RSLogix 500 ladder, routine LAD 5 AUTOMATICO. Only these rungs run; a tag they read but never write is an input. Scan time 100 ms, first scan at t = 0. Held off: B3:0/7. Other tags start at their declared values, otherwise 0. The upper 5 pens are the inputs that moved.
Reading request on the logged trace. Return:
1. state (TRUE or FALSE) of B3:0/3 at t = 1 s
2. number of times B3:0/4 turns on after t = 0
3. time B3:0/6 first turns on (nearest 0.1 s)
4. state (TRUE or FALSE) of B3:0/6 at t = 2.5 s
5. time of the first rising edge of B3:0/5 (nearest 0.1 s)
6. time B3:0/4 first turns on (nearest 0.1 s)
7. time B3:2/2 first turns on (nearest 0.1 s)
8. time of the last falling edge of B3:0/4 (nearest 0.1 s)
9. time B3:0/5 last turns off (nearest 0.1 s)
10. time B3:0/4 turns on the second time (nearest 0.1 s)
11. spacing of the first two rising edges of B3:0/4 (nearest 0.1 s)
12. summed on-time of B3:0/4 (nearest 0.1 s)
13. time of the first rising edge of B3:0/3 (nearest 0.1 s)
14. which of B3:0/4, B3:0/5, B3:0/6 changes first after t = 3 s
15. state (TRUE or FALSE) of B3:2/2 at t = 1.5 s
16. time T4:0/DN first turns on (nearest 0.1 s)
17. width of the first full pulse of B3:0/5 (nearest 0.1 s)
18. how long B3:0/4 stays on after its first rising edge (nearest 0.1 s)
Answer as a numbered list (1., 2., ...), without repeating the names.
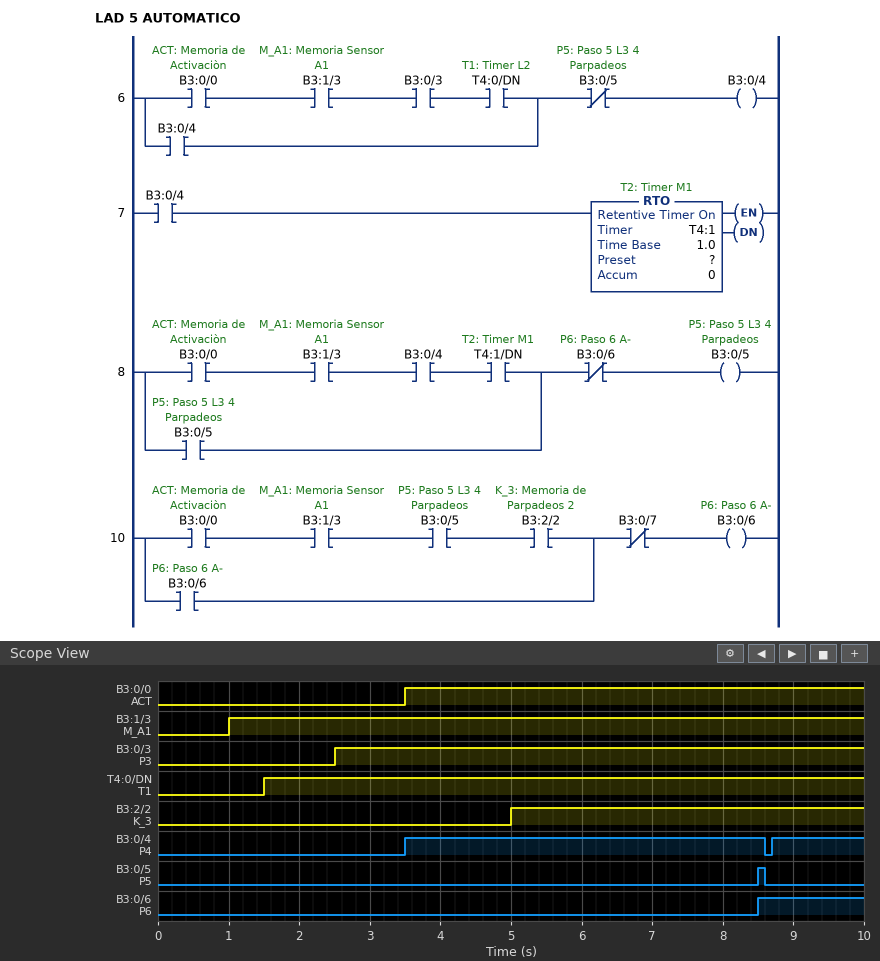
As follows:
1. FALSE
2. 2
3. 8.5 s
4. FALSE
5. 8.5 s
6. 3.5 s
7. 5.0 s
8. 8.6 s
9. 8.6 s
10. 8.7 s
11. 5.2 s
12. 6.4 s
13. 2.5 s
14. B3:0/4
15. FALSE
16. 1.5 s
17. 0.1 s
18. 5.1 s
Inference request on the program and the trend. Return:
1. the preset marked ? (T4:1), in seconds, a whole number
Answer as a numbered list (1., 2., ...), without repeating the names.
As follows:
1. 5 s
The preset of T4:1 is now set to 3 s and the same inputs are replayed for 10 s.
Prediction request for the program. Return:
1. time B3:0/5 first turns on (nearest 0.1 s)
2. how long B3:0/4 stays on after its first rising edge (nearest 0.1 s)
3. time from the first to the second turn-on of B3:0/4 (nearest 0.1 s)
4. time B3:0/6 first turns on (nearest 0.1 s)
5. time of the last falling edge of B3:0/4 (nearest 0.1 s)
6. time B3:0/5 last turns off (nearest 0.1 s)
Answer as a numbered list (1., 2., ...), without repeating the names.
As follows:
1. 6.5 s
2. 3.1 s
3. 3.2 s
4. 6.5 s
5. 6.6 s
6. 6.6 s
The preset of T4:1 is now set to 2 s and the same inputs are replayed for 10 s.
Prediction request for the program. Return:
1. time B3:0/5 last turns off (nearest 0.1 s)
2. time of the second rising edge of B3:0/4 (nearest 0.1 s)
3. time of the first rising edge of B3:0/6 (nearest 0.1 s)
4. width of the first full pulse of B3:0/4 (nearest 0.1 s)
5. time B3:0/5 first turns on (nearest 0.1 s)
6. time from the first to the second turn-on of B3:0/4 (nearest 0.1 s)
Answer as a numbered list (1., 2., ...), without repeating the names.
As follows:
1. 5.6 s
2. 5.7 s
3. 5.5 s
4. 2.1 s
5. 5.5 s
6. 2.2 s
